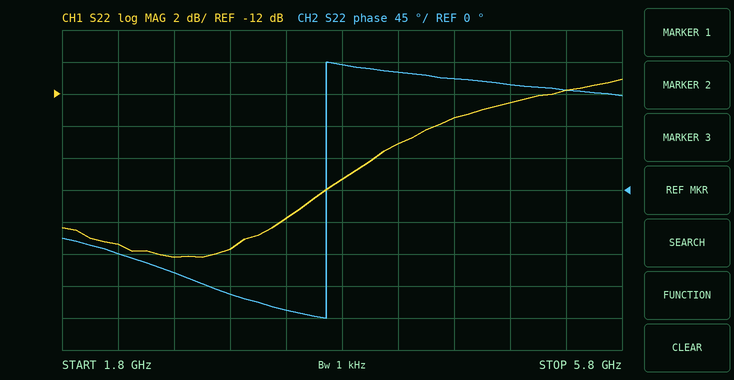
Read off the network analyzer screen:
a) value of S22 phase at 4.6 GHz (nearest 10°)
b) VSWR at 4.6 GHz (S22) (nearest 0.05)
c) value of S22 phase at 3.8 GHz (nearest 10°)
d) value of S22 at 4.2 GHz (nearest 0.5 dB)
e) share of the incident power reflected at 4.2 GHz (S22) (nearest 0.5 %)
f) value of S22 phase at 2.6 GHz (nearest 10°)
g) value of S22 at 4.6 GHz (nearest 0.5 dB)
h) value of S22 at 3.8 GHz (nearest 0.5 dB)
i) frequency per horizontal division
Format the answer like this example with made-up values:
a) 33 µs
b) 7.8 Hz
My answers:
a) 160°
b) 1.55
c) 180°
d) -15.0 dB
e) 3.0 %
f) -120°
g) -13.5 dB
h) -17.5 dB
i) 400 MHz
